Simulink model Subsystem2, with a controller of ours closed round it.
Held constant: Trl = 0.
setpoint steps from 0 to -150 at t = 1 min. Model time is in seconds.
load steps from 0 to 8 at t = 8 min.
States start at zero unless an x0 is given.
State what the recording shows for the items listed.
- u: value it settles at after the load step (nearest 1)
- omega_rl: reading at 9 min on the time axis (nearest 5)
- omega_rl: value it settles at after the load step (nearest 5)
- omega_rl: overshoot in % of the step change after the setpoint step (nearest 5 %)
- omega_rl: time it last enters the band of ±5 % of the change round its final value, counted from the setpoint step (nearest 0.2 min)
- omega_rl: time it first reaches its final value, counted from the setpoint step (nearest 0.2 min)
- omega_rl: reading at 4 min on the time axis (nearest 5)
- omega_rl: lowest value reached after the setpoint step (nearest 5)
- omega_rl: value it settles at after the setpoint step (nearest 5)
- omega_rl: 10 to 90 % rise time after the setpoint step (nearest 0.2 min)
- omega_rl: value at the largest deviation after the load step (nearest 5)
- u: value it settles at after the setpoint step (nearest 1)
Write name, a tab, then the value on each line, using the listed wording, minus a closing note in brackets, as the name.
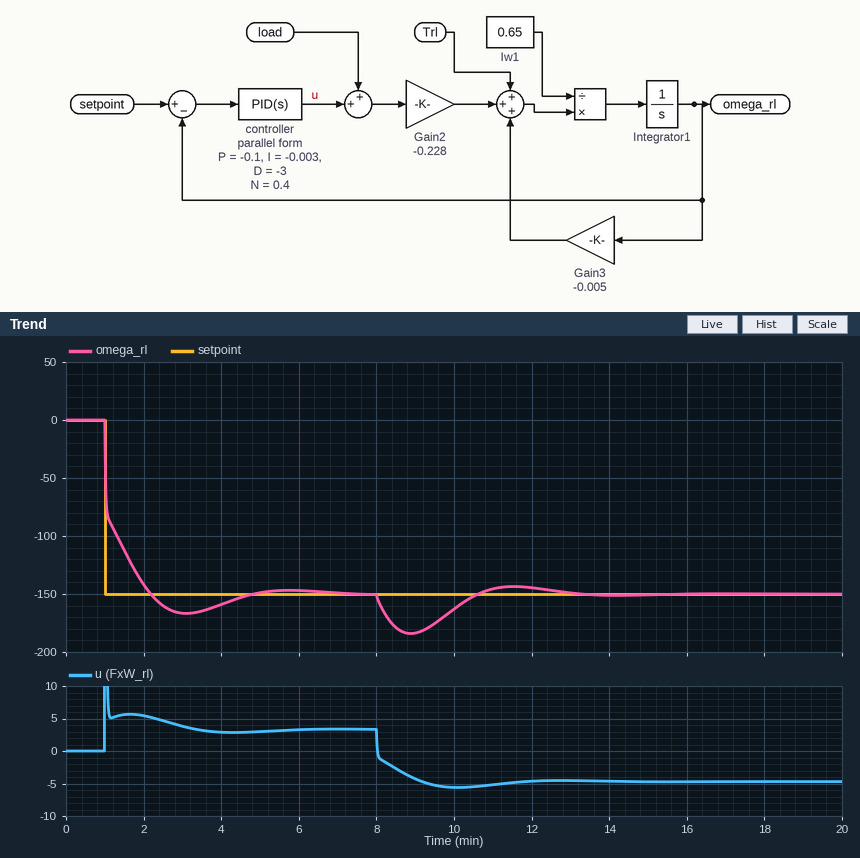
u: value it settles at after the load step	-5
omega_rl: reading at 9 min on the time axis	-185
omega_rl: value it settles at after the load step	-150
omega_rl: overshoot in % of the step change after the setpoint step	10 %
omega_rl: time it last enters the band of ±5 % of the change round its final value, counted from the setpoint step	3.2 min
omega_rl: time it first reaches its final value, counted from the setpoint step	1.2 min
omega_rl: reading at 4 min on the time axis	-160
omega_rl: lowest value reached after the setpoint step	-165
omega_rl: value it settles at after the setpoint step	-150
omega_rl: 10 to 90 % rise time after the setpoint step	0.8 min
omega_rl: value at the largest deviation after the load step	-185
u: value it settles at after the setpoint step	3
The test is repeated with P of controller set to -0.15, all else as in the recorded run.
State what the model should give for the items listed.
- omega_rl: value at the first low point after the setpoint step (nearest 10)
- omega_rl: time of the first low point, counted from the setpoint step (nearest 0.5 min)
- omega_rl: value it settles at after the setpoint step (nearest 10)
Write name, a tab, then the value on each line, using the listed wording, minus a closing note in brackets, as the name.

omega_rl: value at the first low point after the setpoint step	-160
omega_rl: time of the first low point, counted from the setpoint step	2.0 min
omega_rl: value it settles at after the setpoint step	-150
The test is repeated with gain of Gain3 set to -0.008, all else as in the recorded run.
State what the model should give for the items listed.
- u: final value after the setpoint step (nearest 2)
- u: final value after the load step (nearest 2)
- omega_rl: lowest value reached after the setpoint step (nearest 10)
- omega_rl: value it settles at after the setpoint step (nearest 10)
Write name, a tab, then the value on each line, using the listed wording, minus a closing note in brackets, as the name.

u: final value after the setpoint step	6
u: final value after the load step	-2
omega_rl: lowest value reached after the setpoint step	-160
omega_rl: value it settles at after the setpoint step	-150
